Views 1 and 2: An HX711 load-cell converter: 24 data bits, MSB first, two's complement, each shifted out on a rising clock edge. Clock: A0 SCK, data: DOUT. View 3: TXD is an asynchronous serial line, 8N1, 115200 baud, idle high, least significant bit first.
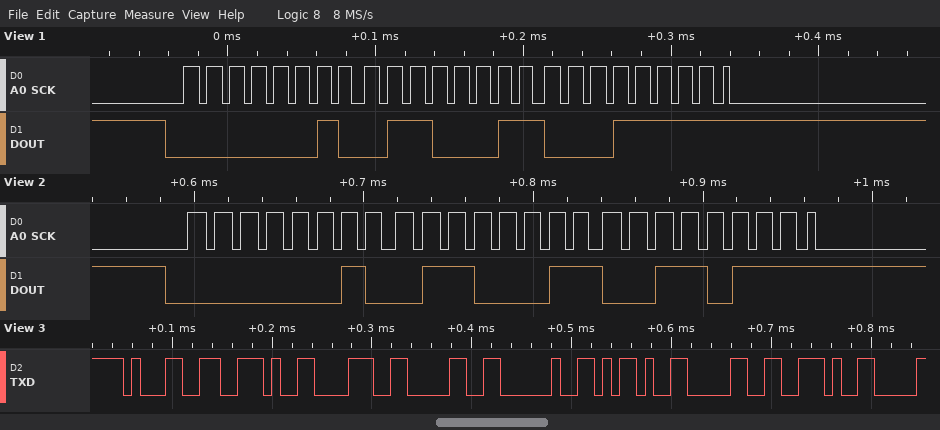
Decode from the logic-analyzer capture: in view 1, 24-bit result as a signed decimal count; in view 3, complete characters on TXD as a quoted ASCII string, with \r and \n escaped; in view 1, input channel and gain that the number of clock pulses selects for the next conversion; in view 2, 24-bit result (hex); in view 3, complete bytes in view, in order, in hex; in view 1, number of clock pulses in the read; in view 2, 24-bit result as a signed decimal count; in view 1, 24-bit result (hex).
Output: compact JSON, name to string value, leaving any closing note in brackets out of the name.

{"in view 1, 24-bit result as a signed decimal count": "156447", "in view 3, complete characters on TXD as a quoted ASCII string, with \\r and \\n escaped": "\"1.80 -0.\"", "in view 1, input channel and gain that the number of clock pulses selects for the next conversion": "channel A, gain 128", "in view 2, 24-bit result": "0x026337", "in view 3, complete bytes in view, in order, in hex": "31 2E 38 30 20 2D 30 2E", "in view 1, number of clock pulses in the read": "25", "in view 2, 24-bit result as a signed decimal count": "156471", "in view 1, 24-bit result": "0x02631F"}
